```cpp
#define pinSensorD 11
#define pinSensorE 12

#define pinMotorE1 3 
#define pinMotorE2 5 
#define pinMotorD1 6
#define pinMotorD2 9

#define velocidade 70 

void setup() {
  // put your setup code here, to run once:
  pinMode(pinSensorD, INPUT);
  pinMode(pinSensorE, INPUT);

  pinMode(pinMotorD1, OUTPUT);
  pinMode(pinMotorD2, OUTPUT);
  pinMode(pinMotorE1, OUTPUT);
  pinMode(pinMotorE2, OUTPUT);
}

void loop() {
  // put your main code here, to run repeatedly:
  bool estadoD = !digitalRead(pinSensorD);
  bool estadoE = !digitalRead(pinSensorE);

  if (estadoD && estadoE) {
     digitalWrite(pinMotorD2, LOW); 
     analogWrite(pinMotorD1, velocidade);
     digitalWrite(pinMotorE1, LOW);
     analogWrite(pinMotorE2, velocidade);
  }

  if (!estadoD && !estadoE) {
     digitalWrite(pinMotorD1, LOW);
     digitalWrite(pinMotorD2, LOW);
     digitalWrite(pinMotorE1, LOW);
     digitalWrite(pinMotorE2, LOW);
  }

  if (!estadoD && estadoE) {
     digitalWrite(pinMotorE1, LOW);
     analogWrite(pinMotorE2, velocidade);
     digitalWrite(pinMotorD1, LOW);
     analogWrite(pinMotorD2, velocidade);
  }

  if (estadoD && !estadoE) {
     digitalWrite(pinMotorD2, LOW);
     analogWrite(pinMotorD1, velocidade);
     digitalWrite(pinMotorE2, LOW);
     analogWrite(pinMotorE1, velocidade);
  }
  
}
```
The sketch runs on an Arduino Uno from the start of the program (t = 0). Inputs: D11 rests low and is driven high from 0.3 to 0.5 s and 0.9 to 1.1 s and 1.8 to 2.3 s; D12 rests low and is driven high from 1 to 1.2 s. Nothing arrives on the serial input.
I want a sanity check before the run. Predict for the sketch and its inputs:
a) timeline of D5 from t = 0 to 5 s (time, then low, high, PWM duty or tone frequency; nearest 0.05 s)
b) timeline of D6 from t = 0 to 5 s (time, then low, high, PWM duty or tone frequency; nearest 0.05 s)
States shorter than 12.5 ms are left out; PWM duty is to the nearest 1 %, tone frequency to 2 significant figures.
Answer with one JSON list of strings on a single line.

["0 s PWM 28 %; 1 s low; 1.2 s PWM 28 %", "0 s PWM 28 %; 0.3 s low; 0.5 s PWM 28 %; 0.9 s low; 1.1 s PWM 28 %; 1.8 s low; 2.3 s PWM 28 %"]
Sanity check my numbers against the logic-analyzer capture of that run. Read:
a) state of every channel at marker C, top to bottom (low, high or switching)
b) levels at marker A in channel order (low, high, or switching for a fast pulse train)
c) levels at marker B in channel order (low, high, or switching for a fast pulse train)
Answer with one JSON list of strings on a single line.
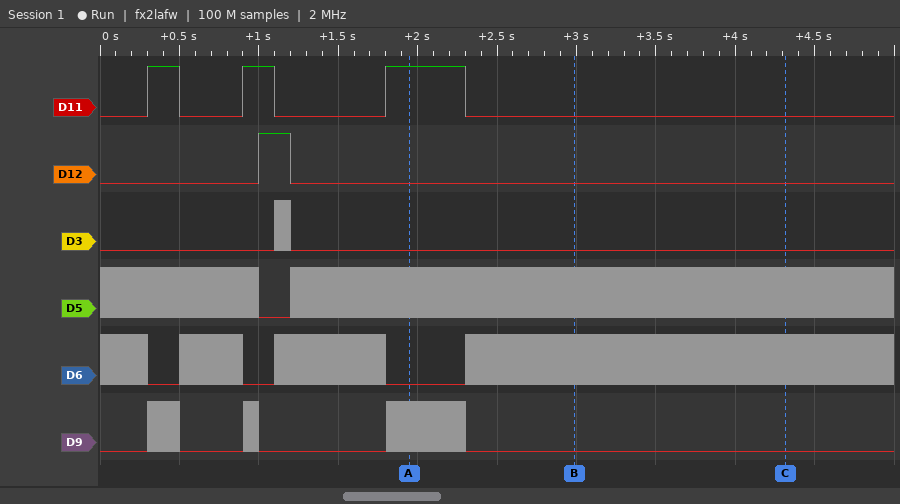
["D11 low, D12 low, D3 low, D5 switching, D6 switching, D9 low", "D11 high, D12 low, D3 low, D5 switching, D6 low, D9 switching", "D11 low, D12 low, D3 low, D5 switching, D6 switching, D9 low"]
